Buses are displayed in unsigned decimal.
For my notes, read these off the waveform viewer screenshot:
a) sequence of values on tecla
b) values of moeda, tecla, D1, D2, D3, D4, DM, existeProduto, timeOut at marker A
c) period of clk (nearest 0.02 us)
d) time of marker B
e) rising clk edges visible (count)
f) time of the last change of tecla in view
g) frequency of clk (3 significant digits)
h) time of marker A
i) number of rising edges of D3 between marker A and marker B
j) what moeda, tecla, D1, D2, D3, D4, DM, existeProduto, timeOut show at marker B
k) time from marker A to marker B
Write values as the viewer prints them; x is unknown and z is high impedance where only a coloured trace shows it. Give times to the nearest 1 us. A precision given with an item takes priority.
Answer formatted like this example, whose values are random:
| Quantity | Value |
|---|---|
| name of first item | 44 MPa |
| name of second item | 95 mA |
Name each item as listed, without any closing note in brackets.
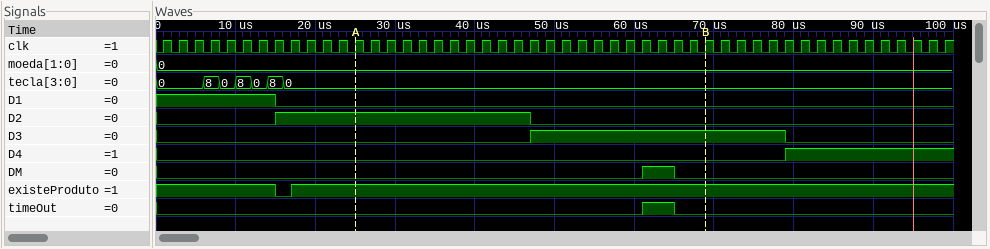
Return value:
| Quantity | Value |
|---|---|
| sequence of values on tecla | 0, 8, 0, 8, 0, 8, 0 |
| values of moeda, tecla, D1, D2, D3, D4, DM, existeProduto, timeOut at marker A | moeda=0, tecla=0, D1=0, D2=1, D3=0, D4=0, DM=0, existeProduto=1, timeOut=0 |
| period of clk | 2 us |
| time of marker B | 69 us |
| rising clk edges visible | 50 |
| time of the last change of tecla in view | 16 us |
| frequency of clk | 500 kHz |
| time of marker A | 25 us |
| number of rising edges of D3 between marker A and marker B | 1 |
| what moeda, tecla, D1, D2, D3, D4, DM, existeProduto, timeOut show at marker B | moeda=0, tecla=0, D1=0, D2=0, D3=1, D4=0, DM=0, existeProduto=1, timeOut=0 |
| time from marker A to marker B | 44 us |
